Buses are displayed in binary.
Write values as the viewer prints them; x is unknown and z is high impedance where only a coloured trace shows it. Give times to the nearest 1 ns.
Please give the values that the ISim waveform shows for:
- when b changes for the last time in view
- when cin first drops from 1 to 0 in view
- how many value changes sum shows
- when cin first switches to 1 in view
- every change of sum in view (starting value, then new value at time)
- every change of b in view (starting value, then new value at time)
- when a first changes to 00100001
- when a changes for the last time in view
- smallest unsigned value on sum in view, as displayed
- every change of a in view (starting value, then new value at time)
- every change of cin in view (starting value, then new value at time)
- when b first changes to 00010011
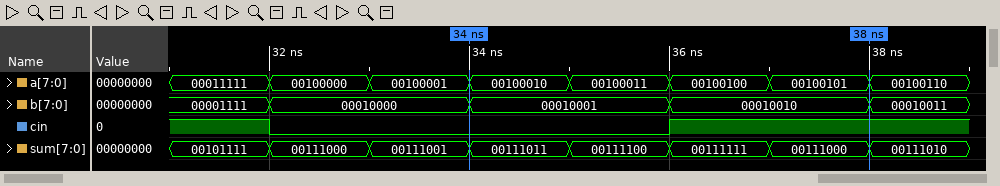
38 ns
32 ns
7
36 ns
00101111, 00111000 at 32 ns, 00111001 at 33 ns, 00111011 at 34 ns, 00111100 at 35 ns, 00111111 at 36 ns, 00111000 at 37 ns, 00111010 at 38 ns
00001111, 00010000 at 32 ns, 00010001 at 34 ns, 00010010 at 36 ns, 00010011 at 38 ns
33 ns
38 ns
00101111
00011111, 00100000 at 32 ns, 00100001 at 33 ns, 00100010 at 34 ns, 00100011 at 35 ns, 00100100 at 36 ns, 00100101 at 37 ns, 00100110 at 38 ns
1, 0 at 32 ns, 1 at 36 ns
38 ns
